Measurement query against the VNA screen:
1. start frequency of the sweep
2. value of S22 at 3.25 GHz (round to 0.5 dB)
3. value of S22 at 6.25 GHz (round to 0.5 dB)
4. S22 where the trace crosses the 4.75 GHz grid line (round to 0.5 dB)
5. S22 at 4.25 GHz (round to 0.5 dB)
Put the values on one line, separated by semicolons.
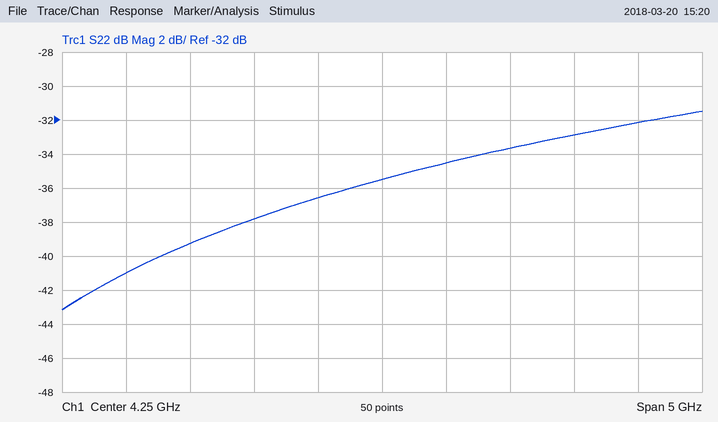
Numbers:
1.75 GHz; -38.0 dB; -32.0 dB; -34.5 dB; -35.5 dB
